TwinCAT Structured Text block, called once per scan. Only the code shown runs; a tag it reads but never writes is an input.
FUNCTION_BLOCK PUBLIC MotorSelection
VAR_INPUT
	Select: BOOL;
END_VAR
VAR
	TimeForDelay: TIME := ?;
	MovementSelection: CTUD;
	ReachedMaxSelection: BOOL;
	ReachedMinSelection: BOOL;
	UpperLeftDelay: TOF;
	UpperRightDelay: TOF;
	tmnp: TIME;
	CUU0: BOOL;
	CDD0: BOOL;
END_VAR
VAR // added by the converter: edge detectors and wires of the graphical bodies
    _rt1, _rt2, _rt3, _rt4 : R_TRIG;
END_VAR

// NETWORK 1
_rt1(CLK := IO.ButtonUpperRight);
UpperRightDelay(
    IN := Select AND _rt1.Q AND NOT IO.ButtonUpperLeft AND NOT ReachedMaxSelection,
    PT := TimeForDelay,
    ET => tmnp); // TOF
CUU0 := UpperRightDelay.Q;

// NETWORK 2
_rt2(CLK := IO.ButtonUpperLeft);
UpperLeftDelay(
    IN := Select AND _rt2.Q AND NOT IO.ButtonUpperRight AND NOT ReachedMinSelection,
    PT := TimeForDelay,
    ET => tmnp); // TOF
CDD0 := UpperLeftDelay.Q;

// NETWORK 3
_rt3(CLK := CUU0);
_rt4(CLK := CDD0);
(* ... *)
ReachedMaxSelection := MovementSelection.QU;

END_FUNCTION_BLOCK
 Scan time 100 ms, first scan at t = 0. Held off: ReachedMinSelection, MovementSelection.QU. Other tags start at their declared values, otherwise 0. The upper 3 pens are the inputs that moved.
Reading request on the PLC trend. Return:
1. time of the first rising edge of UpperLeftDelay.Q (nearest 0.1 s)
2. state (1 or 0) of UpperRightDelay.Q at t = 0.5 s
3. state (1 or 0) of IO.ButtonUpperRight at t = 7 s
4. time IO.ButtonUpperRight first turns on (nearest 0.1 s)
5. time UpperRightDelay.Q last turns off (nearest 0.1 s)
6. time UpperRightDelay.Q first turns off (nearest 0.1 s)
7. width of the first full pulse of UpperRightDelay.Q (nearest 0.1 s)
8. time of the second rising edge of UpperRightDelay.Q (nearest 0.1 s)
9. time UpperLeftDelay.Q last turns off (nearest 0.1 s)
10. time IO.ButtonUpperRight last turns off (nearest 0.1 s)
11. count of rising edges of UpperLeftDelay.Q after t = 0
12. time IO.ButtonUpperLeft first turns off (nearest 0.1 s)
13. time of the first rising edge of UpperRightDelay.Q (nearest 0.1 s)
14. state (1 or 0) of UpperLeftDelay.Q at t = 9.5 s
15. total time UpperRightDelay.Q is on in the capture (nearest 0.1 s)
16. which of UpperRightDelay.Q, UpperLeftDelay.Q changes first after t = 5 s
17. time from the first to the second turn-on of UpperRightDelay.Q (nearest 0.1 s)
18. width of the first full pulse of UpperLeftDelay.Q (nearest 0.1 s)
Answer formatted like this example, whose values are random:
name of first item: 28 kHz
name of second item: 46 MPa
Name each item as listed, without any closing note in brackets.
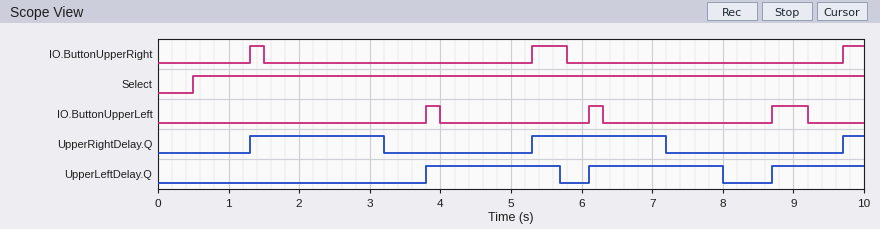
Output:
time of the first rising edge of UpperLeftDelay.Q: 3.8 s
state (1 or 0) of UpperRightDelay.Q at t = 0.5 s: 0
state (1 or 0) of IO.ButtonUpperRight at t = 7 s: 0
time IO.ButtonUpperRight first turns on: 1.3 s
time UpperRightDelay.Q last turns off: 7.2 s
time UpperRightDelay.Q first turns off: 3.2 s
width of the first full pulse of UpperRightDelay.Q: 1.9 s
time of the second rising edge of UpperRightDelay.Q: 5.3 s
time UpperLeftDelay.Q last turns off: 8.0 s
time IO.ButtonUpperRight last turns off: 5.8 s
count of rising edges of UpperLeftDelay.Q after t = 0: 3
time IO.ButtonUpperLeft first turns off: 4.0 s
time of the first rising edge of UpperRightDelay.Q: 1.3 s
state (1 or 0) of UpperLeftDelay.Q at t = 9.5 s: 1
total time UpperRightDelay.Q is on in the capture: 4.1 s
which of UpperRightDelay.Q, UpperLeftDelay.Q changes first after t = 5 s: UpperRightDelay.Q
time from the first to the second turn-on of UpperRightDelay.Q: 4.0 s
width of the first full pulse of UpperLeftDelay.Q: 1.9 s
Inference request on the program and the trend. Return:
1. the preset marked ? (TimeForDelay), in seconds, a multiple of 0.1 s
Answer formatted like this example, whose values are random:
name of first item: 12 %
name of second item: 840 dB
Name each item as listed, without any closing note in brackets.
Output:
the preset marked ? (TimeForDelay), in seconds, a multiple of 0.1 s: 1.8 s
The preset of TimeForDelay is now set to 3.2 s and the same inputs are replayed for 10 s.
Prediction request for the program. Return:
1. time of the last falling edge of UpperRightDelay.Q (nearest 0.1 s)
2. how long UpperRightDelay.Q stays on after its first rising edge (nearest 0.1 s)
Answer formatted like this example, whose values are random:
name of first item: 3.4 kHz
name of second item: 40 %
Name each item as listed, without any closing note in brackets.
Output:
time of the last falling edge of UpperRightDelay.Q: 8.6 s
how long UpperRightDelay.Q stays on after its first rising edge: 3.3 s
